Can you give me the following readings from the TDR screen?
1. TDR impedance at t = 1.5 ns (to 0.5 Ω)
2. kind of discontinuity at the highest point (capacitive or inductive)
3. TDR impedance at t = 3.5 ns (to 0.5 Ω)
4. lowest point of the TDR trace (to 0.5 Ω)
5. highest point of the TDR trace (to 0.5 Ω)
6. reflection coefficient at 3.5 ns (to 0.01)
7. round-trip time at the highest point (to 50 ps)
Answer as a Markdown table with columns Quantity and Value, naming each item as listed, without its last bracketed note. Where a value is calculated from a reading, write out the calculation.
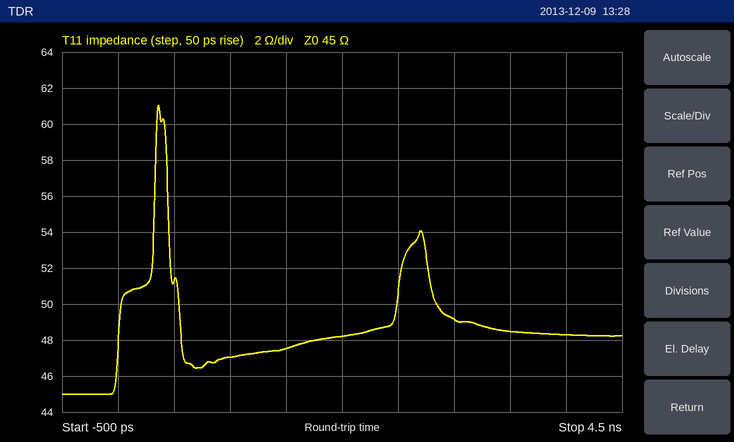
| Quantity | Value |
|---|---|
| TDR impedance at t = 1.5 ns | 47.5 Ω |
| kind of discontinuity at the highest point | inductive |
| TDR impedance at t = 3.5 ns | 48.5 Ω |
| lowest point of the TDR trace | 45.0 Ω |
| highest point of the TDR trace | 61.0 Ω |
| reflection coefficient at 3.5 ns | (48.5 − 45)/(48.5 + 45) ≈ +0.04 |
| round-trip time at the highest point | 350 ps |
